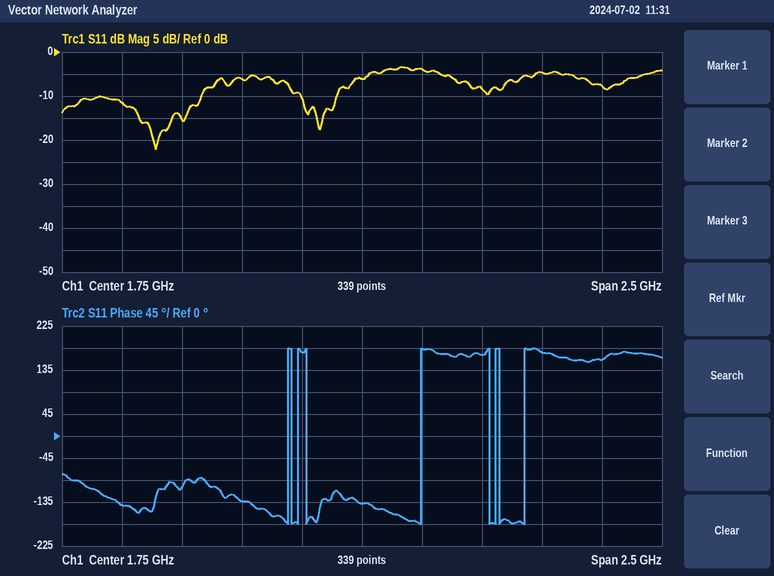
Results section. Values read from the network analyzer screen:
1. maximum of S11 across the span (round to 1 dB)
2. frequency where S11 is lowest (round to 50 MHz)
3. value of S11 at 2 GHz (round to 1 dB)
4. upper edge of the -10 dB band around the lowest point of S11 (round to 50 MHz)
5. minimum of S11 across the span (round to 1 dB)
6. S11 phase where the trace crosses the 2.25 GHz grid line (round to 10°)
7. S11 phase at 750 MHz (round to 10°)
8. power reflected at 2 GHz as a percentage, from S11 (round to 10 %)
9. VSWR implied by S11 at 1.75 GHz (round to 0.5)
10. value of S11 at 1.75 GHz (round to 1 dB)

-3 dB
900 MHz
-4 dB
1.10 GHz
-22 dB
170°
-140°
40 %
3.0
-6 dB
